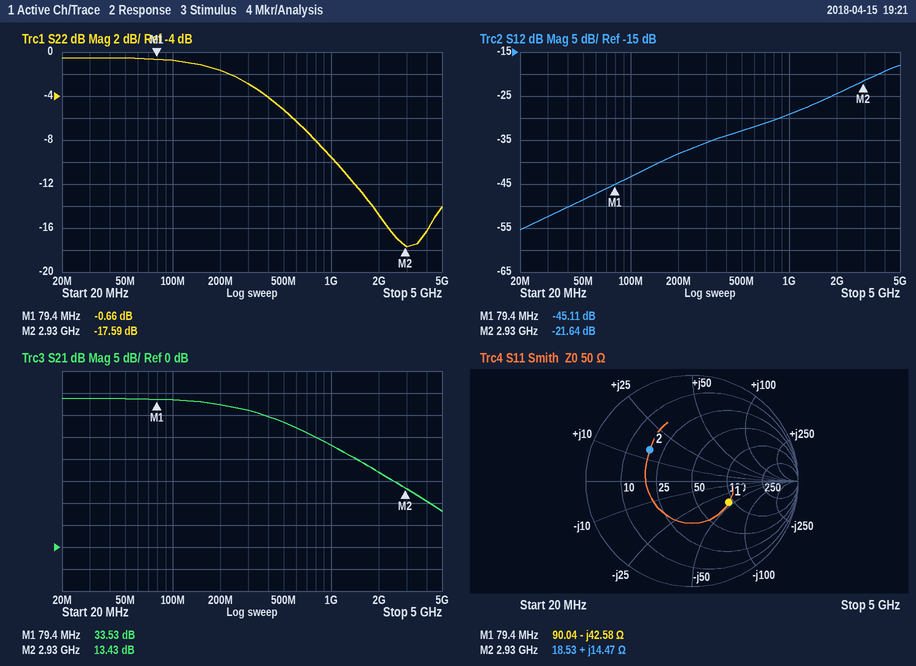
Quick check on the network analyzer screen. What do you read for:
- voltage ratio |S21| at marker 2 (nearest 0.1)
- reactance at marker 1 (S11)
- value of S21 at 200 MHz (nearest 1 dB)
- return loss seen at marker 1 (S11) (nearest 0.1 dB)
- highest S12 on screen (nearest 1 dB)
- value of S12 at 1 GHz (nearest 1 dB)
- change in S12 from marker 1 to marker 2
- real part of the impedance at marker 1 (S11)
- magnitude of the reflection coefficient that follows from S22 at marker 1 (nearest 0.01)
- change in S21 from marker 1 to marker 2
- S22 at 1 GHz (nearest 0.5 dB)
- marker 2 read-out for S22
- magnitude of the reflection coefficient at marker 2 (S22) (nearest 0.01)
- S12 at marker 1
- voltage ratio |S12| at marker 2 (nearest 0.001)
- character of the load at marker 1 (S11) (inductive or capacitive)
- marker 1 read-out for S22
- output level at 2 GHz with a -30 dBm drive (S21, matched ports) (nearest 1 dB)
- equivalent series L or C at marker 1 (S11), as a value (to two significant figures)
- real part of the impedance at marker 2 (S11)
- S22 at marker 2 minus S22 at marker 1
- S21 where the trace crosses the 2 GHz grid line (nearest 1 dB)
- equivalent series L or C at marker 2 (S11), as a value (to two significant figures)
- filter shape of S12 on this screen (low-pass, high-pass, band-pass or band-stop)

4.7
-42.58 Ω
32 dB
8.0 dB
-18 dB
-29 dB
23.47 dB
90.04 Ω
0.93
-20.10 dB
-9.5 dB
-17.59 dB
0.13
-45.11 dB
0.083
capacitive
-0.66 dB
-13 dBm
47 pF
18.53 Ω
-16.93 dB
17 dB
790 pH
high-pass
